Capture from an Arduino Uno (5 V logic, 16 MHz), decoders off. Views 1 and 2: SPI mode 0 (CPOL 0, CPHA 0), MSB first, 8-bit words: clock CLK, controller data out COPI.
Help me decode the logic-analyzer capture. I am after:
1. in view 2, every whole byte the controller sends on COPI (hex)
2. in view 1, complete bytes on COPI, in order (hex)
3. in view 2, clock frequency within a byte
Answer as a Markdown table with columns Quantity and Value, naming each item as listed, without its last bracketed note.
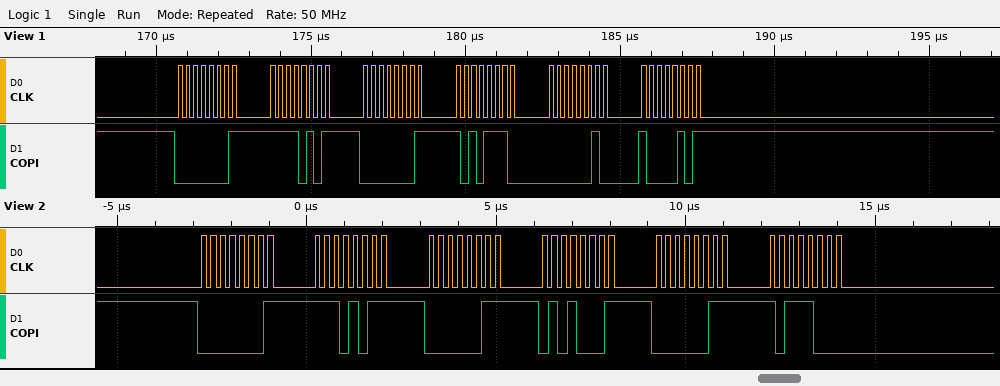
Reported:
| Quantity | Value |
|---|---|
| in view 2, every whole byte the controller sends on COPI | 01 EB 03 51 03 B8 |
| in view 1, complete bytes on COPI, in order | 01 F5 01 AE 02 85 |
| in view 2, clock frequency within a byte | 4 MHz |
